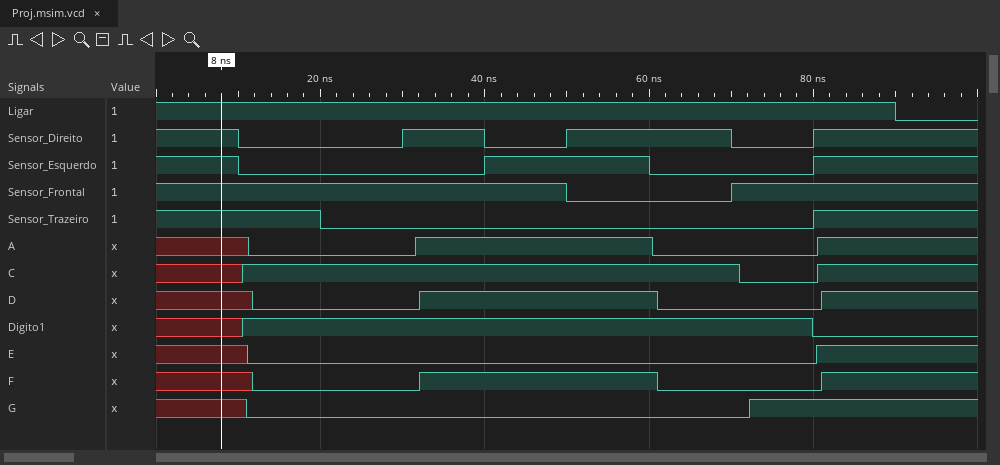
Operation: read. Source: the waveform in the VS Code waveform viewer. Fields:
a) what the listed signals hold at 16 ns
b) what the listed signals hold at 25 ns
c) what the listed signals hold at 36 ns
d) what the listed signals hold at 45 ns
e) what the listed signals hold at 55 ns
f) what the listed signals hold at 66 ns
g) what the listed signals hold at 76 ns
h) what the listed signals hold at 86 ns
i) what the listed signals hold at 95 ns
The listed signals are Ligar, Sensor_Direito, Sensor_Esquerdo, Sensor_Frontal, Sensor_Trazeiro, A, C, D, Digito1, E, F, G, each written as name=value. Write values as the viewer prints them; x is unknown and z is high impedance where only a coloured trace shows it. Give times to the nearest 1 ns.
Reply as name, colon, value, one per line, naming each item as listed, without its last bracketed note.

what the listed signals hold at 16 ns: Ligar=1, Sensor_Direito=0, Sensor_Esquerdo=0, Sensor_Frontal=1, Sensor_Trazeiro=1, A=0, C=1, D=0, Digito1=1, E=0, F=0, G=0
what the listed signals hold at 25 ns: Ligar=1, Sensor_Direito=0, Sensor_Esquerdo=0, Sensor_Frontal=1, Sensor_Trazeiro=0, A=0, C=1, D=0, Digito1=1, E=0, F=0, G=0
what the listed signals hold at 36 ns: Ligar=1, Sensor_Direito=1, Sensor_Esquerdo=0, Sensor_Frontal=1, Sensor_Trazeiro=0, A=1, C=1, D=1, Digito1=1, E=0, F=1, G=0
what the listed signals hold at 45 ns: Ligar=1, Sensor_Direito=0, Sensor_Esquerdo=1, Sensor_Frontal=1, Sensor_Trazeiro=0, A=1, C=1, D=1, Digito1=1, E=0, F=1, G=0
what the listed signals hold at 55 ns: Ligar=1, Sensor_Direito=1, Sensor_Esquerdo=1, Sensor_Frontal=0, Sensor_Trazeiro=0, A=1, C=1, D=1, Digito1=1, E=0, F=1, G=0
what the listed signals hold at 66 ns: Ligar=1, Sensor_Direito=1, Sensor_Esquerdo=0, Sensor_Frontal=0, Sensor_Trazeiro=0, A=0, C=1, D=0, Digito1=1, E=0, F=0, G=0
what the listed signals hold at 76 ns: Ligar=1, Sensor_Direito=0, Sensor_Esquerdo=0, Sensor_Frontal=1, Sensor_Trazeiro=0, A=0, C=0, D=0, Digito1=1, E=0, F=0, G=1
what the listed signals hold at 86 ns: Ligar=1, Sensor_Direito=1, Sensor_Esquerdo=1, Sensor_Frontal=1, Sensor_Trazeiro=1, A=1, C=1, D=1, Digito1=0, E=1, F=1, G=1
what the listed signals hold at 95 ns: Ligar=0, Sensor_Direito=1, Sensor_Esquerdo=1, Sensor_Frontal=1, Sensor_Trazeiro=1, A=1, C=1, D=1, Digito1=0, E=1, F=1, G=1
